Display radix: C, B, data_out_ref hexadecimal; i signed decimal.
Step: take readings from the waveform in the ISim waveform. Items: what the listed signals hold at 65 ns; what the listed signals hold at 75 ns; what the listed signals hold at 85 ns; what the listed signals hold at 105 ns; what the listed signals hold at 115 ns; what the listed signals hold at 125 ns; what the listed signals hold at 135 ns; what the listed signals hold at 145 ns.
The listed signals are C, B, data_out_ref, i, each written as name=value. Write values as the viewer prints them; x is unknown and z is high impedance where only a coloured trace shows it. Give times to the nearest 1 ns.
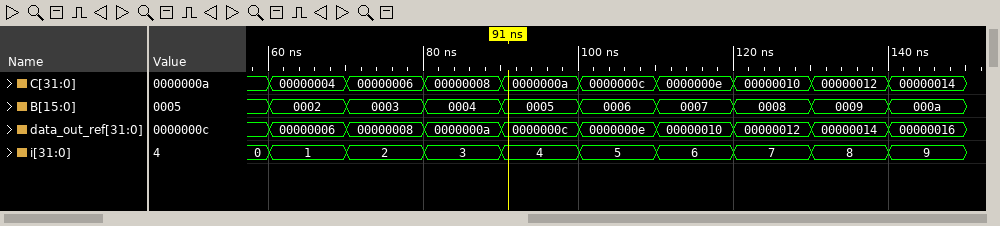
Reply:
C=00000004, B=0002, data_out_ref=00000006, i=1
C=00000006, B=0003, data_out_ref=00000008, i=2
C=00000008, B=0004, data_out_ref=0000000a, i=3
C=0000000c, B=0006, data_out_ref=0000000e, i=5
C=0000000e, B=0007, data_out_ref=00000010, i=6
C=00000010, B=0008, data_out_ref=00000012, i=7
C=00000012, B=0009, data_out_ref=00000014, i=8
C=00000014, B=000a, data_out_ref=00000016, i=9
